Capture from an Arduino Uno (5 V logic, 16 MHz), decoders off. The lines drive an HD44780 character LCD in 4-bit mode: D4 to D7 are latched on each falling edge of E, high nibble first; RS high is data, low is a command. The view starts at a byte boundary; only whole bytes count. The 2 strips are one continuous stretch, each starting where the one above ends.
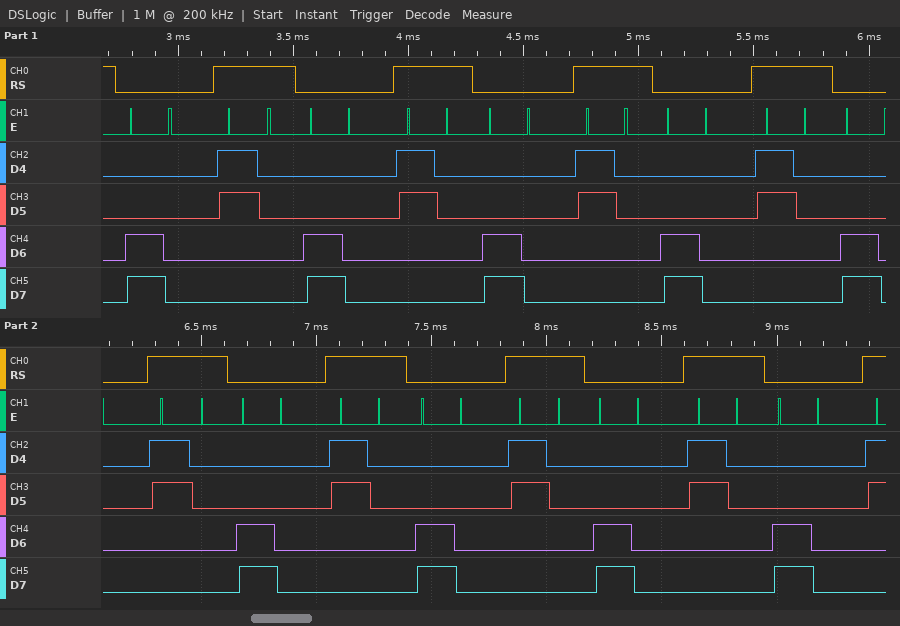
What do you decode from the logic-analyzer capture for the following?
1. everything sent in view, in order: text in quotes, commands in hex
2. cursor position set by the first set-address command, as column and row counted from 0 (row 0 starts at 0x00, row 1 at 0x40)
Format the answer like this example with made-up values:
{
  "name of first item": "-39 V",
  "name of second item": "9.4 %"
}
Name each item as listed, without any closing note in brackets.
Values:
{
  "everything sent in view, in order: text in quotes, commands in hex": "0xC0 \"0\" 0xC0 \"0\" 0xC0 \"0\" 0xC0 \"0\" 0xC0 \"0\" 0xC0 \"0\" 0xC0 \"0\" 0xC0 \"0\" 0xC0",
  "cursor position set by the first set-address command, as column and row counted from 0": "column 0, row 1"
}
